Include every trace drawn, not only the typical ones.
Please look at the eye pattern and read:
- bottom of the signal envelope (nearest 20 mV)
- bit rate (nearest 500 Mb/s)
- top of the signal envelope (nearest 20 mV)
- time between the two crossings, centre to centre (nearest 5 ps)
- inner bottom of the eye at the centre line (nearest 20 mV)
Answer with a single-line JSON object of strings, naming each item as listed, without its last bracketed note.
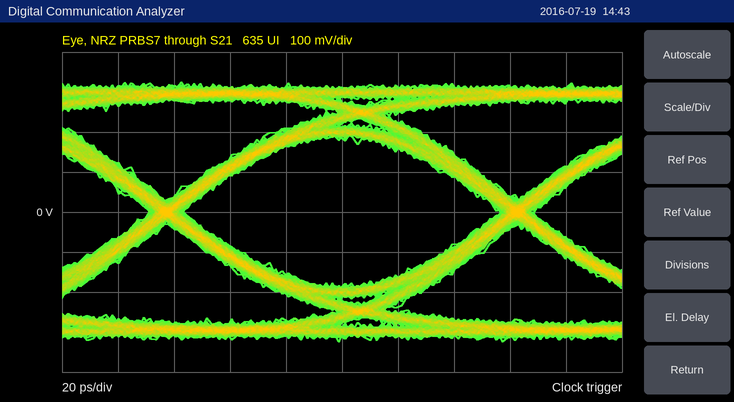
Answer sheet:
{"bottom of the signal envelope": "-320 mV", "bit rate": "8.0 Gb/s", "top of the signal envelope": "320 mV", "time between the two crossings, centre to centre": "125 ps", "inner bottom of the eye at the centre line": "-180 mV"}
